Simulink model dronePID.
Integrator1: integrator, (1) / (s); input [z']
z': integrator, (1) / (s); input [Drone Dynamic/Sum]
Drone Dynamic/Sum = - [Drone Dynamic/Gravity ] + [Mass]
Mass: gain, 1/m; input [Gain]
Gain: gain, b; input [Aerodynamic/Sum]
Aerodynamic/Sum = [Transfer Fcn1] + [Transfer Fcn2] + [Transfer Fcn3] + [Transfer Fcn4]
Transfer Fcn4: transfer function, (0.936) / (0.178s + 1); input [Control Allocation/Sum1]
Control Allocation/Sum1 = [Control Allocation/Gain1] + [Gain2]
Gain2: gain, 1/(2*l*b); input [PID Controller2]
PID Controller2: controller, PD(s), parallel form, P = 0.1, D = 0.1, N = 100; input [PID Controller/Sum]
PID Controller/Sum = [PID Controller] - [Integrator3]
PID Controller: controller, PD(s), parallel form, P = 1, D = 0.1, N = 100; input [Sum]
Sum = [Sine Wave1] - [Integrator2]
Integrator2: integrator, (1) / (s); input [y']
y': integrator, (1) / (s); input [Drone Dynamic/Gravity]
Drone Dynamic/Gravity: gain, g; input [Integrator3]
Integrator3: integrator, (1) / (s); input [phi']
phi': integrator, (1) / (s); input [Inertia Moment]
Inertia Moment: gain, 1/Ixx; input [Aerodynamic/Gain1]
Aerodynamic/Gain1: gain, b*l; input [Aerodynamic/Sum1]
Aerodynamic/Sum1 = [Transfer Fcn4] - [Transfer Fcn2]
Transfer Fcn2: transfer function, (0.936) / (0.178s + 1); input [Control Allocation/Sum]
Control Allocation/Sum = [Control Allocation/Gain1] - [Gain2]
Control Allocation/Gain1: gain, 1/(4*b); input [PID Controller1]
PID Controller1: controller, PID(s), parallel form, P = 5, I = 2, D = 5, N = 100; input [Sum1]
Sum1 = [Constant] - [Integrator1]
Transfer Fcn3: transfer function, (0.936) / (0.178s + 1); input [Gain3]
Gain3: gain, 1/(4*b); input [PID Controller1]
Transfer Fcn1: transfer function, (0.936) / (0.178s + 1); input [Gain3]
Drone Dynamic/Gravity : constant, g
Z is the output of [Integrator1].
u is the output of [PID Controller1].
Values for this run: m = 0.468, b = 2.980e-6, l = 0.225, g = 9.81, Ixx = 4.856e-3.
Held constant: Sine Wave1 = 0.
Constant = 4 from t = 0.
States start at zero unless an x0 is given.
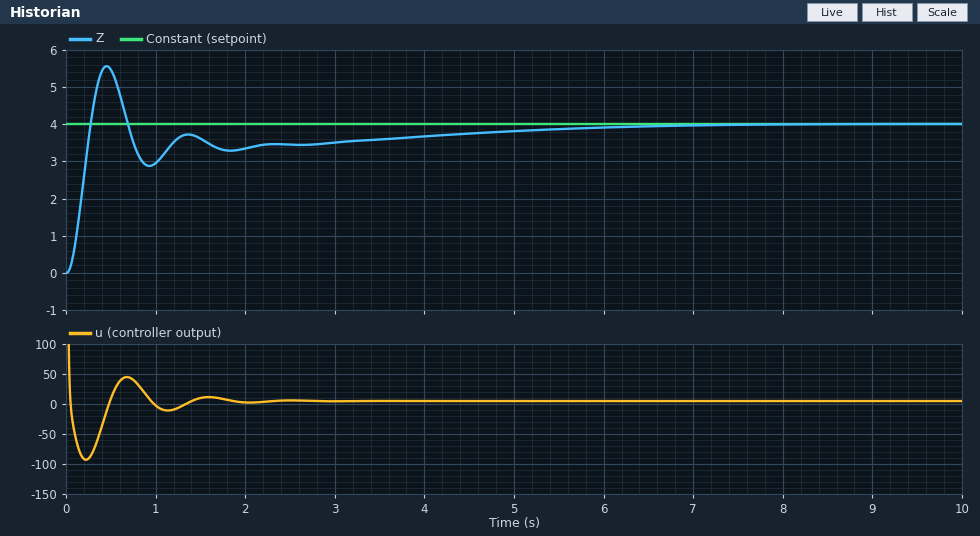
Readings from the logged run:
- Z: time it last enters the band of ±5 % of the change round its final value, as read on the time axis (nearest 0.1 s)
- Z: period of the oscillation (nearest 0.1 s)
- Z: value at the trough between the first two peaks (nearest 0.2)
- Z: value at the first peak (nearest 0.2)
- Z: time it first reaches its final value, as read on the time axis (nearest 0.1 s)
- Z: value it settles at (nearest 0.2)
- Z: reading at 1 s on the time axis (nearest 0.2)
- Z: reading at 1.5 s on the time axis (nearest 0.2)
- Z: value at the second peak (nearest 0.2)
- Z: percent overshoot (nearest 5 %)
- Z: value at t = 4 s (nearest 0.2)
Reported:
4.9 s
0.9 s
2.8
5.6
0.3 s
4.0
3.0
3.6
3.8
40 %
3.6
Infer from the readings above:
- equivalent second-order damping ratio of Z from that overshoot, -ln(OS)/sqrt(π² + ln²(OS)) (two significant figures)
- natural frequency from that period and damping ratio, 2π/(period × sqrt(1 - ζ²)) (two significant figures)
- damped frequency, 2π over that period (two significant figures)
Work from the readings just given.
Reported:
0.28
7.3 rad/s
7.0 rad/s
